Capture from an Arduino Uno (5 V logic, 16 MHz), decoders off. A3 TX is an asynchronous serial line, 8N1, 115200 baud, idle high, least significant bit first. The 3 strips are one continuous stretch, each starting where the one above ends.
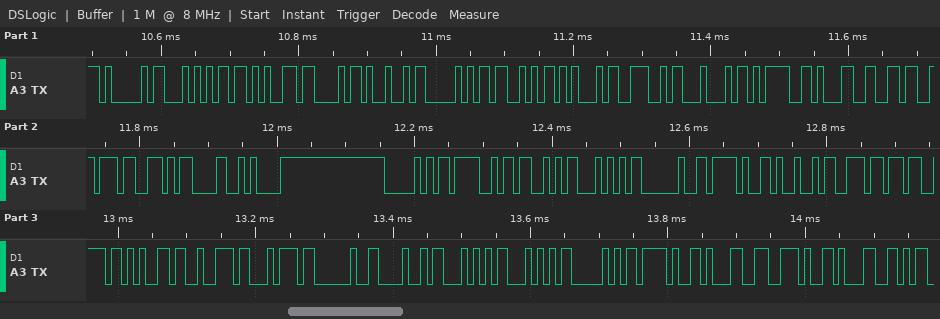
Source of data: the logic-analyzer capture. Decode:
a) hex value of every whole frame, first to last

41 54 2B 43 49 50 53 45 4E 44 3D 31 36 37 0D 0A 50 4F 53 54 20 2F 49 6E 73 65 72 74 20 48 54 54 50 2F 31 2E 31
